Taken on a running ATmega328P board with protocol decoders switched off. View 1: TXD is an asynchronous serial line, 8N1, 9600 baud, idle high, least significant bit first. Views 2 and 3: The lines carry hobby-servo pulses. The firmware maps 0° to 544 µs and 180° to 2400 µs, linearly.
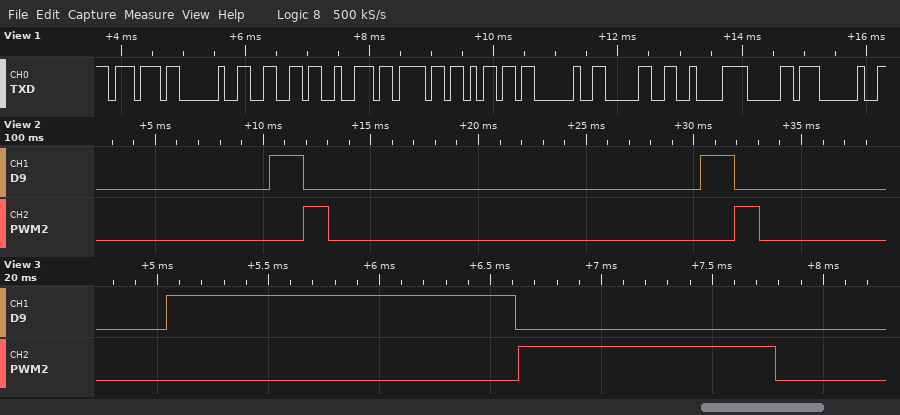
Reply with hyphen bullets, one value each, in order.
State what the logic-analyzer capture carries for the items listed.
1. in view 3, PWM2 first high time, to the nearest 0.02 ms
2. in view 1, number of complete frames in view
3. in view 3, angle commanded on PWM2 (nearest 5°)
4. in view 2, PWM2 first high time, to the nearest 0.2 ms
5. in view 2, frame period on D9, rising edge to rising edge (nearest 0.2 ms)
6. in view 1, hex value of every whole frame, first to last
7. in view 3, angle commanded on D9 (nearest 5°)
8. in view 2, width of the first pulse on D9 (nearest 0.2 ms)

- 1.16 ms
- 11
- 60°
- 1.2 ms
- 20.0 ms
- 77 20 66 72 6F 6D 20 30 C2 B0 20
- 100°
- 1.6 ms
